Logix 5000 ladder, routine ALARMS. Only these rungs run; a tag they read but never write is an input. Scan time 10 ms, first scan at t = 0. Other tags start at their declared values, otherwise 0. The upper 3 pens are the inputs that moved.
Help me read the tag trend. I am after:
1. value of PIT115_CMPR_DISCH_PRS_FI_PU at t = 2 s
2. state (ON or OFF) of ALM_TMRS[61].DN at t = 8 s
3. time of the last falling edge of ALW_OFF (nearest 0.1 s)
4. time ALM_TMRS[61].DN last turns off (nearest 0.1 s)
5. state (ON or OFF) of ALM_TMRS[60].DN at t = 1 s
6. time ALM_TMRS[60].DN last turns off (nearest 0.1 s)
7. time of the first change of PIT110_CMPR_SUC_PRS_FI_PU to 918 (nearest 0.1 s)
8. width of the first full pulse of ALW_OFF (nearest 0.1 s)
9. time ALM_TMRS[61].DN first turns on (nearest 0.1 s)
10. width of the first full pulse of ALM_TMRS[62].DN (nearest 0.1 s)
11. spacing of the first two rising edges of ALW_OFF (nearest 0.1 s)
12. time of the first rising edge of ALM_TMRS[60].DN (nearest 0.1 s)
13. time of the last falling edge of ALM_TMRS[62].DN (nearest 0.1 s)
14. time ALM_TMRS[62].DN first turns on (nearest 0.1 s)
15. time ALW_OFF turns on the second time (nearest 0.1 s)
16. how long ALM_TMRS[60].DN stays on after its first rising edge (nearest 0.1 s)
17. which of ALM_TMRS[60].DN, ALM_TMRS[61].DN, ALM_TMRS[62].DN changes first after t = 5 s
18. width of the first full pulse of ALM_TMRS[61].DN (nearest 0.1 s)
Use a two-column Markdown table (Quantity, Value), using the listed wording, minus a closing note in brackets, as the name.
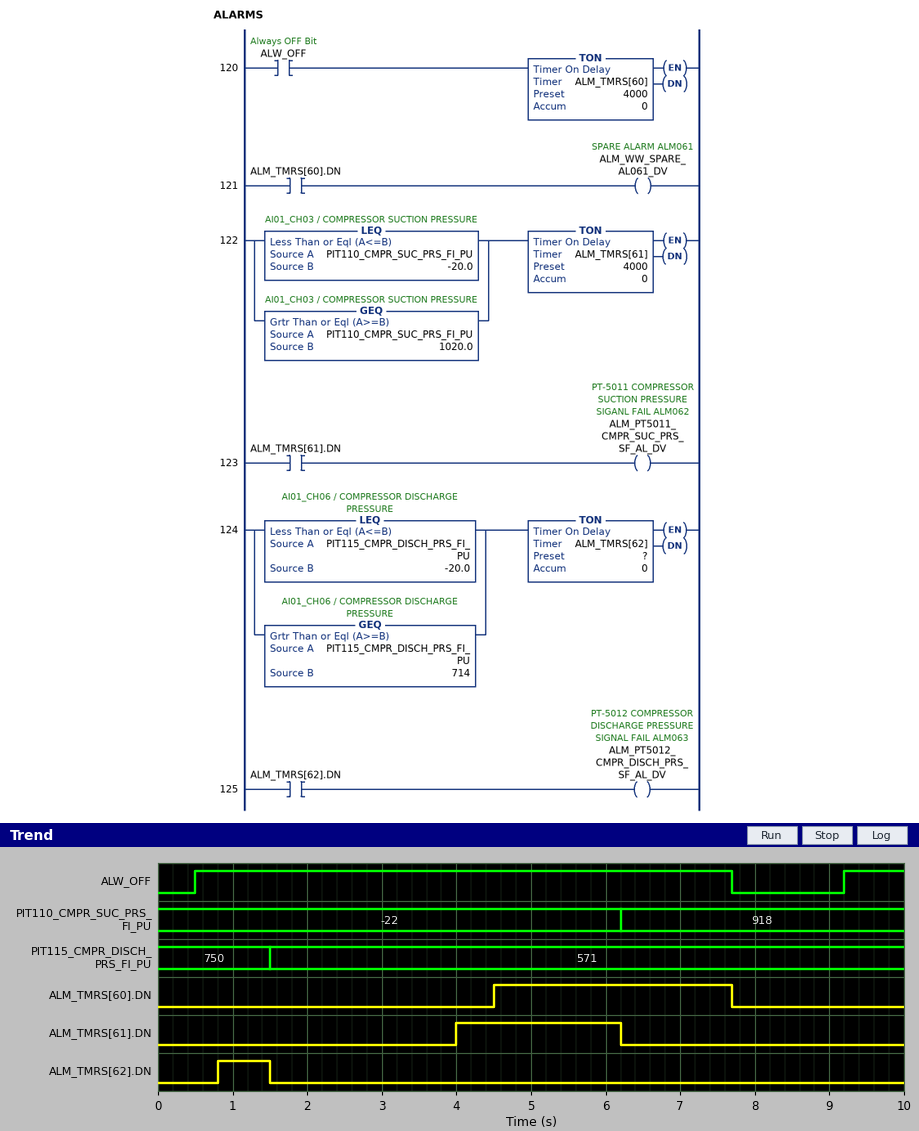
| Quantity | Value |
|---|---|
| value of PIT115_CMPR_DISCH_PRS_FI_PU at t = 2 s | 571 |
| state (ON or OFF) of ALM_TMRS[61].DN at t = 8 s | OFF |
| time of the last falling edge of ALW_OFF | 7.7 s |
| time ALM_TMRS[61].DN last turns off | 6.2 s |
| state (ON or OFF) of ALM_TMRS[60].DN at t = 1 s | OFF |
| time ALM_TMRS[60].DN last turns off | 7.7 s |
| time of the first change of PIT110_CMPR_SUC_PRS_FI_PU to 918 | 6.2 s |
| width of the first full pulse of ALW_OFF | 7.2 s |
| time ALM_TMRS[61].DN first turns on | 4.0 s |
| width of the first full pulse of ALM_TMRS[62].DN | 0.7 s |
| spacing of the first two rising edges of ALW_OFF | 8.7 s |
| time of the first rising edge of ALM_TMRS[60].DN | 4.5 s |
| time of the last falling edge of ALM_TMRS[62].DN | 1.5 s |
| time ALM_TMRS[62].DN first turns on | 0.8 s |
| time ALW_OFF turns on the second time | 9.2 s |
| how long ALM_TMRS[60].DN stays on after its first rising edge | 3.2 s |
| which of ALM_TMRS[60].DN, ALM_TMRS[61].DN, ALM_TMRS[62].DN changes first after t = 5 s | ALM_TMRS[61].DN |
| width of the first full pulse of ALM_TMRS[61].DN | 2.2 s |
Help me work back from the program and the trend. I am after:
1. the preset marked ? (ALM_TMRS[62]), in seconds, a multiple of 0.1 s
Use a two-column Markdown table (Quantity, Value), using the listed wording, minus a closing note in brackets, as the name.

| Quantity | Value |
|---|---|
| the preset marked ? (ALM_TMRS[62]), in seconds, a multiple of 0.1 s | 0.8 s |
